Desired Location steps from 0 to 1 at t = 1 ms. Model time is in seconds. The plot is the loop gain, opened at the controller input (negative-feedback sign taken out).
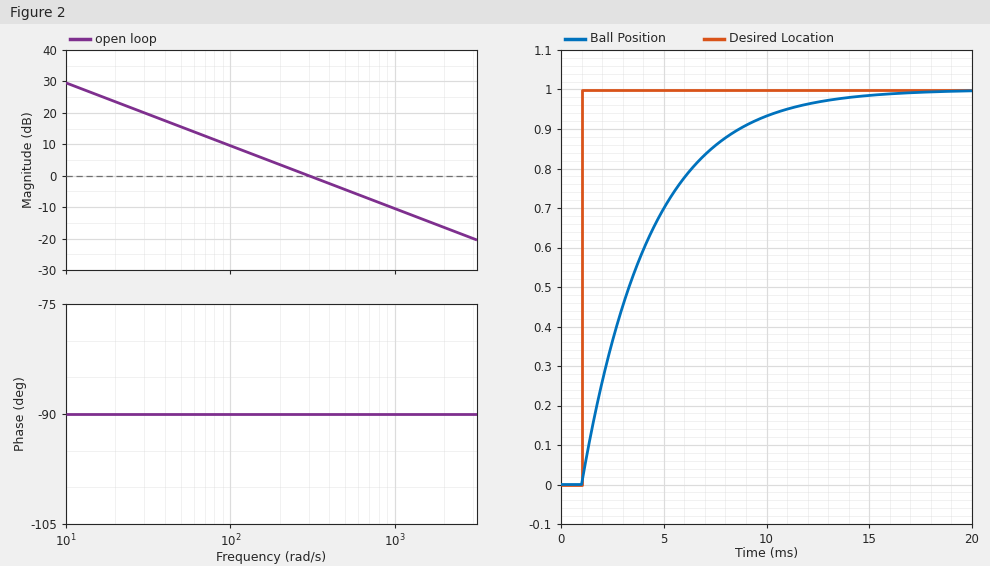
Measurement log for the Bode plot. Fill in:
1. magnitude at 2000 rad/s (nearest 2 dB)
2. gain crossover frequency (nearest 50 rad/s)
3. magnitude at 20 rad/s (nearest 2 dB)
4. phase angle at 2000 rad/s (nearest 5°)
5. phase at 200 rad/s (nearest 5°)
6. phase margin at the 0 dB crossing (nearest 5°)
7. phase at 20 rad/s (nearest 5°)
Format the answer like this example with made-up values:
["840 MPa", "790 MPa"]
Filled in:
["-16 dB", "300 rad/s", "24 dB", "-90°", "-90°", "90°", "-90°"]
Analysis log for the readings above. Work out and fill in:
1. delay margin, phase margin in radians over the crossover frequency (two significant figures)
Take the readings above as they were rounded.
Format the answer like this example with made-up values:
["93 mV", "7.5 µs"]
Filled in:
["0.0052 s"]
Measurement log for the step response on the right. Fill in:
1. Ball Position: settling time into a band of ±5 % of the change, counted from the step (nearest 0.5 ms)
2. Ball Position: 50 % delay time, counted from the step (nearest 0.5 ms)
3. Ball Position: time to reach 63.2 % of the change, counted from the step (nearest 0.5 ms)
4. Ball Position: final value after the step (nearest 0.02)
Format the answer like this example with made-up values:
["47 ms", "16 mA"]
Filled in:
["10.0 ms", "2.5 ms", "3.5 ms", "1.00"]
